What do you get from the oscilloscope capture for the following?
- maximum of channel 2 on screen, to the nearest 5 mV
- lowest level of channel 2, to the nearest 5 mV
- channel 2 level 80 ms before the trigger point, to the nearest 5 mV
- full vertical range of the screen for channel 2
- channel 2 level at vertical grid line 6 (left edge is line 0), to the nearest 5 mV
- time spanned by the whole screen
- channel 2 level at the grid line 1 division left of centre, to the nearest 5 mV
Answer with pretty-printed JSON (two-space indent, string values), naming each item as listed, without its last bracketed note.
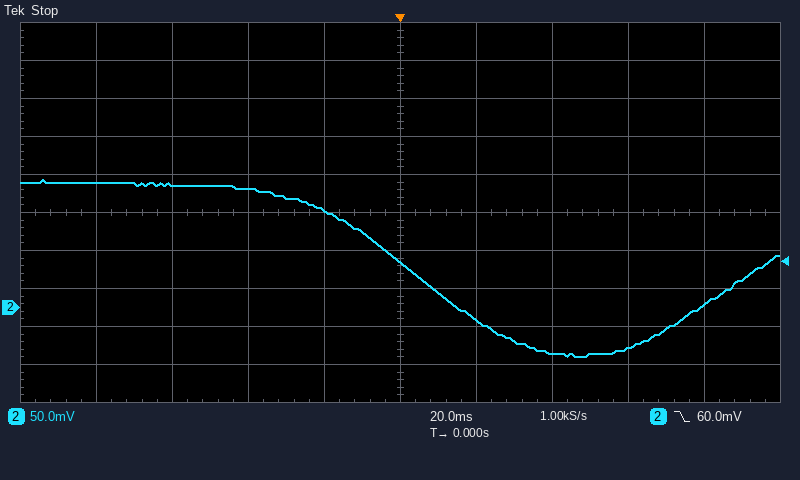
{
  "maximum of channel 2 on screen, to the nearest 5 mV": "170 mV",
  "lowest level of channel 2, to the nearest 5 mV": "-65 mV",
  "channel 2 level 80 ms before the trigger point, to the nearest 5 mV": "165 mV",
  "full vertical range of the screen for channel 2": "500 mV",
  "channel 2 level at vertical grid line 6 (left edge is line 0), to the nearest 5 mV": "-15 mV",
  "time spanned by the whole screen": "200 ms",
  "channel 2 level at the grid line 1 division left of centre, to the nearest 5 mV": "130 mV"
}
